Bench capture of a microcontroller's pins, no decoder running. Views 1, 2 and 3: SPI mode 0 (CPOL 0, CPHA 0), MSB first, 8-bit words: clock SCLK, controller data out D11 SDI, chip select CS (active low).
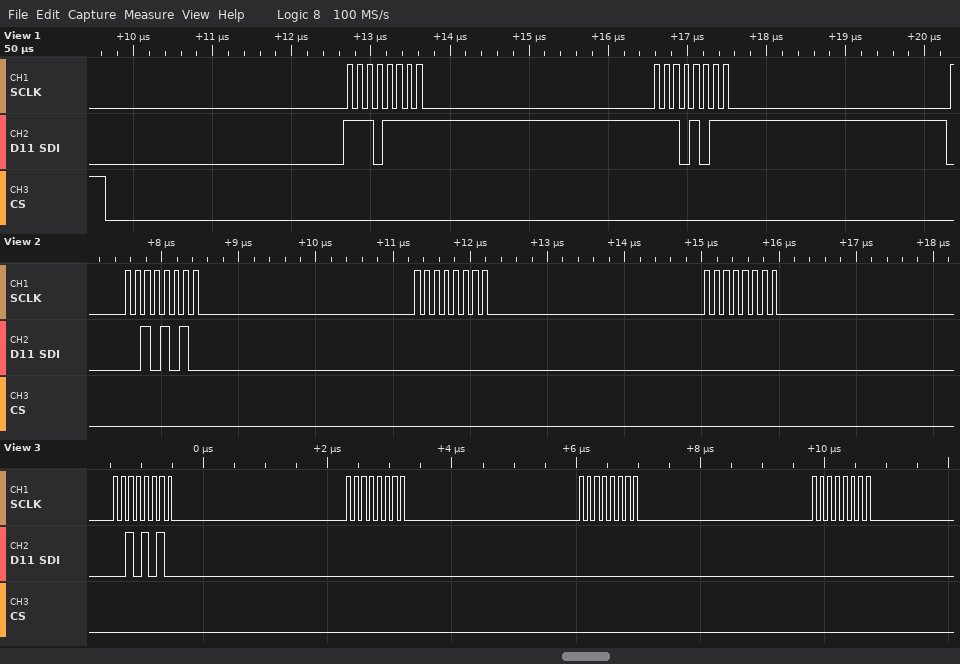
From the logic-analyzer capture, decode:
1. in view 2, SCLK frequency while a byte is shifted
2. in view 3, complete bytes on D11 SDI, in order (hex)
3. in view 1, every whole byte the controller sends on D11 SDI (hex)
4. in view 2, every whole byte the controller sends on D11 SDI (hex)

8 MHz
2A 00 00 00
0xEF 0xEB
2A 00 00
